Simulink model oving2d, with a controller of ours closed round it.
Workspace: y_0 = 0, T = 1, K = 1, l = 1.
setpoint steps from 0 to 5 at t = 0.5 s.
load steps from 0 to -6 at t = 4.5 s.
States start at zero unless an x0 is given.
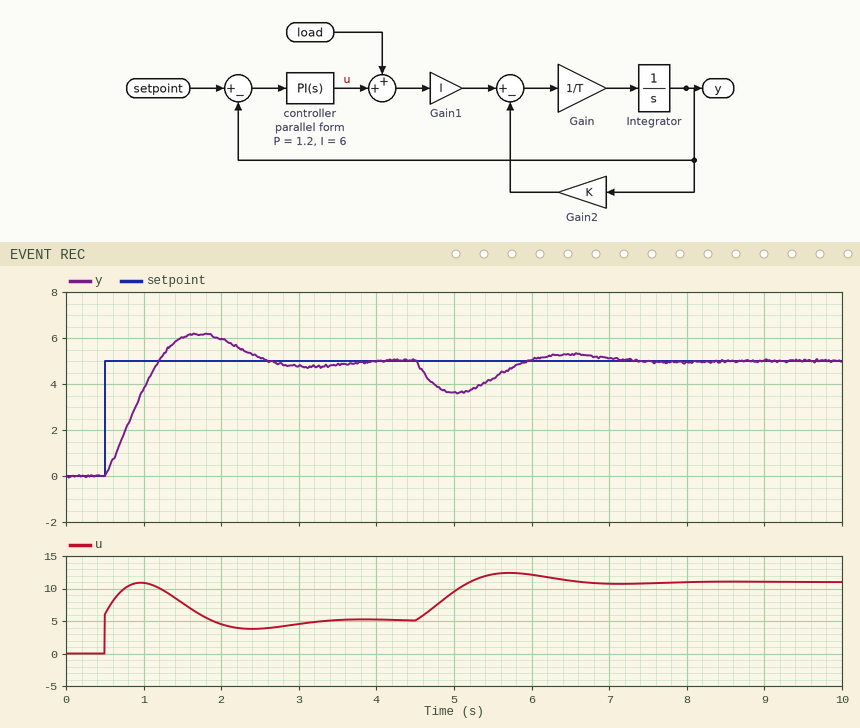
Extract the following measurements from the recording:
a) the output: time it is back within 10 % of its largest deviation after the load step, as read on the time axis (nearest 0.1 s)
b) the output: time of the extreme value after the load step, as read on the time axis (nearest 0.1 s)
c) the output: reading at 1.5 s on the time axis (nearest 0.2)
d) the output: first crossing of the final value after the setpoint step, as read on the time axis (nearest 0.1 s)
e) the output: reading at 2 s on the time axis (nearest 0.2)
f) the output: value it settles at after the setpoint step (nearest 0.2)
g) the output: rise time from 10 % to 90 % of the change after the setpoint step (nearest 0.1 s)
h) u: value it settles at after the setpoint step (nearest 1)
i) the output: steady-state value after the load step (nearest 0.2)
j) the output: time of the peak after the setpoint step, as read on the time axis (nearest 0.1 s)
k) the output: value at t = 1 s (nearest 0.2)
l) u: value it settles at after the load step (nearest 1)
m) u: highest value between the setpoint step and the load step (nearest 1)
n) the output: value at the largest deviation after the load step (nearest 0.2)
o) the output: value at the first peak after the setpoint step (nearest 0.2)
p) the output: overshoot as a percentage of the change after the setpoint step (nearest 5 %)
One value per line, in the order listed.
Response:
7.0 s
5.0 s
6.0
1.2 s
6.0
5.0
0.5 s
5
5.0
1.7 s
3.8
11
11
3.6
6.2
25 %
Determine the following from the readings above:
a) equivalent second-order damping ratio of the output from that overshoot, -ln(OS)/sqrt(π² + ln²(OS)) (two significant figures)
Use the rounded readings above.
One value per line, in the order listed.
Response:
0.40
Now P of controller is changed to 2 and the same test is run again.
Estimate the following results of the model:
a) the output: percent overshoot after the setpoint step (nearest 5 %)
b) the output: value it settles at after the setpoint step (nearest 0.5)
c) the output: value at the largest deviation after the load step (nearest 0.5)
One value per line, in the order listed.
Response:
15 %
5.0
4.0
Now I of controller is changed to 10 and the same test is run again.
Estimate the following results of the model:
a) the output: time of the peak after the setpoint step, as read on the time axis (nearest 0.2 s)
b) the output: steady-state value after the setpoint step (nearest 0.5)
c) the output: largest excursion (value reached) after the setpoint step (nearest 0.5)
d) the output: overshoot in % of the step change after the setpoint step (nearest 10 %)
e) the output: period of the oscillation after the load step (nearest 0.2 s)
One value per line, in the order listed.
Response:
1.4 s
5.0
6.5
30 %
2.2 s
